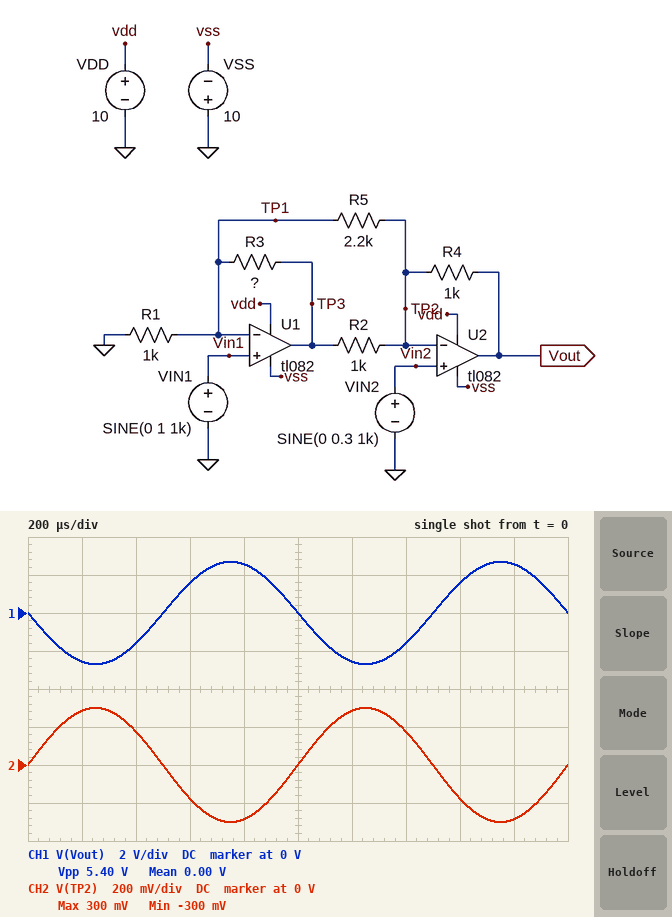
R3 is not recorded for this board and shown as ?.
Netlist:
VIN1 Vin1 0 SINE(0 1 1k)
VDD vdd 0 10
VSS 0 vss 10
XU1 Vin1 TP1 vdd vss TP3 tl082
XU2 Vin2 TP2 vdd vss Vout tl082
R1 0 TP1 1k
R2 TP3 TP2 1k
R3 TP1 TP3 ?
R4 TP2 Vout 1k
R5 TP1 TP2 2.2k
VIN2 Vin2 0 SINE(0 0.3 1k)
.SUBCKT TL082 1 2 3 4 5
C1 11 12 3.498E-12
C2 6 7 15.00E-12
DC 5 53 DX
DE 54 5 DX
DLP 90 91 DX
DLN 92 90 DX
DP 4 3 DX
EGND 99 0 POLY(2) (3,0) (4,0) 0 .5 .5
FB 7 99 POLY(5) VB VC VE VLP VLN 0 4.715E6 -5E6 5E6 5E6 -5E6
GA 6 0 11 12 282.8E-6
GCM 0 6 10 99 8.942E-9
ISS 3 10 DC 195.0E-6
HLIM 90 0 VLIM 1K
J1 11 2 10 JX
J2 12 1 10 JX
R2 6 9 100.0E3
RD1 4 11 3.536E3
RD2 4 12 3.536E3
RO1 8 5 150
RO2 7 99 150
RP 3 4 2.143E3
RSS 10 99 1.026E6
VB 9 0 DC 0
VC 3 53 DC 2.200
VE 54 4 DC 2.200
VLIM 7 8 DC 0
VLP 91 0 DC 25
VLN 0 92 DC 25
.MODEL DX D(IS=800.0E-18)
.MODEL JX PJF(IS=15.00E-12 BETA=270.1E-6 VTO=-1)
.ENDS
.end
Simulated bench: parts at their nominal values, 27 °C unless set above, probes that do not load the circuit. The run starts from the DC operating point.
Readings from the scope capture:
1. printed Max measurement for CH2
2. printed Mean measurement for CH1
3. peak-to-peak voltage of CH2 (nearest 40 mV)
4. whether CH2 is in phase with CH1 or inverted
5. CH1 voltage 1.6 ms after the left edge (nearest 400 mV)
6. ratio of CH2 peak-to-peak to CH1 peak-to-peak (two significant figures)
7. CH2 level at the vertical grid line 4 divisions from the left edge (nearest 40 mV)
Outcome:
300 mV
0.00 V
600 mV
inverted
1.6 V
0.11
-280 mV
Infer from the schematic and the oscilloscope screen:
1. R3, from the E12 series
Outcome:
1.5 kΩ
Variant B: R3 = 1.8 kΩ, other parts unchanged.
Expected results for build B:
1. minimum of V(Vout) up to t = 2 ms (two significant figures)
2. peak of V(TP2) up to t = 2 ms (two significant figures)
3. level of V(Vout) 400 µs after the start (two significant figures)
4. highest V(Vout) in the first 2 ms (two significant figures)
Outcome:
-3.1 V
300 mV
-1.8 V
3.1 V
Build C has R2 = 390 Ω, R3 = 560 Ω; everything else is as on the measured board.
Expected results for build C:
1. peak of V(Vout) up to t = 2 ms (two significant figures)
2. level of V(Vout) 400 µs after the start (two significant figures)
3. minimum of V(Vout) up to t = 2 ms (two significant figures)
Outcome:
3.7 V
-2.2 V
-3.7 V
